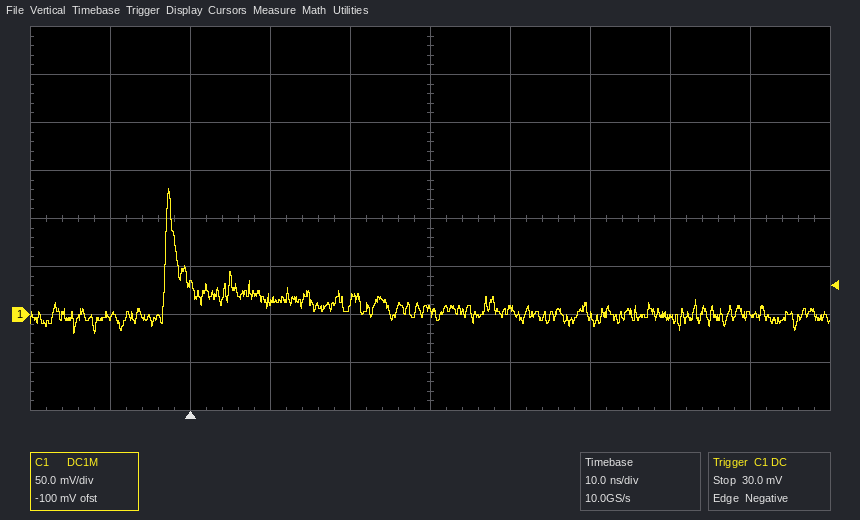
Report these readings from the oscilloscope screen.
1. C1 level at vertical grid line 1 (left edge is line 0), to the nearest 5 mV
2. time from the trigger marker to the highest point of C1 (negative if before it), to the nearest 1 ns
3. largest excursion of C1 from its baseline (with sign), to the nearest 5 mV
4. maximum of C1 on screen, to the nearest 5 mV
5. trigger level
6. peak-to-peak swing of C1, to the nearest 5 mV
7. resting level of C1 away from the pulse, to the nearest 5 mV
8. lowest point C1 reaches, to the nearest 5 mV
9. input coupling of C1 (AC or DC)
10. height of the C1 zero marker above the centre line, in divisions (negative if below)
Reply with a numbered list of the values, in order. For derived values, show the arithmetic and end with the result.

1. 0 mV
2. -3 ns
3. 130 mV − (0 mV) = +130 mV
4. 130 mV
5. 30.0 mV
6. 130 mV − (-20 mV) = 150 mV
7. 0 mV
8. -20 mV
9. DC
10. -2.0 div
